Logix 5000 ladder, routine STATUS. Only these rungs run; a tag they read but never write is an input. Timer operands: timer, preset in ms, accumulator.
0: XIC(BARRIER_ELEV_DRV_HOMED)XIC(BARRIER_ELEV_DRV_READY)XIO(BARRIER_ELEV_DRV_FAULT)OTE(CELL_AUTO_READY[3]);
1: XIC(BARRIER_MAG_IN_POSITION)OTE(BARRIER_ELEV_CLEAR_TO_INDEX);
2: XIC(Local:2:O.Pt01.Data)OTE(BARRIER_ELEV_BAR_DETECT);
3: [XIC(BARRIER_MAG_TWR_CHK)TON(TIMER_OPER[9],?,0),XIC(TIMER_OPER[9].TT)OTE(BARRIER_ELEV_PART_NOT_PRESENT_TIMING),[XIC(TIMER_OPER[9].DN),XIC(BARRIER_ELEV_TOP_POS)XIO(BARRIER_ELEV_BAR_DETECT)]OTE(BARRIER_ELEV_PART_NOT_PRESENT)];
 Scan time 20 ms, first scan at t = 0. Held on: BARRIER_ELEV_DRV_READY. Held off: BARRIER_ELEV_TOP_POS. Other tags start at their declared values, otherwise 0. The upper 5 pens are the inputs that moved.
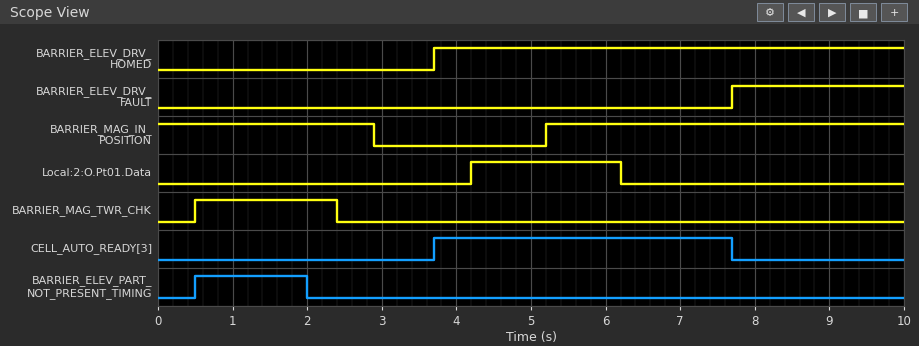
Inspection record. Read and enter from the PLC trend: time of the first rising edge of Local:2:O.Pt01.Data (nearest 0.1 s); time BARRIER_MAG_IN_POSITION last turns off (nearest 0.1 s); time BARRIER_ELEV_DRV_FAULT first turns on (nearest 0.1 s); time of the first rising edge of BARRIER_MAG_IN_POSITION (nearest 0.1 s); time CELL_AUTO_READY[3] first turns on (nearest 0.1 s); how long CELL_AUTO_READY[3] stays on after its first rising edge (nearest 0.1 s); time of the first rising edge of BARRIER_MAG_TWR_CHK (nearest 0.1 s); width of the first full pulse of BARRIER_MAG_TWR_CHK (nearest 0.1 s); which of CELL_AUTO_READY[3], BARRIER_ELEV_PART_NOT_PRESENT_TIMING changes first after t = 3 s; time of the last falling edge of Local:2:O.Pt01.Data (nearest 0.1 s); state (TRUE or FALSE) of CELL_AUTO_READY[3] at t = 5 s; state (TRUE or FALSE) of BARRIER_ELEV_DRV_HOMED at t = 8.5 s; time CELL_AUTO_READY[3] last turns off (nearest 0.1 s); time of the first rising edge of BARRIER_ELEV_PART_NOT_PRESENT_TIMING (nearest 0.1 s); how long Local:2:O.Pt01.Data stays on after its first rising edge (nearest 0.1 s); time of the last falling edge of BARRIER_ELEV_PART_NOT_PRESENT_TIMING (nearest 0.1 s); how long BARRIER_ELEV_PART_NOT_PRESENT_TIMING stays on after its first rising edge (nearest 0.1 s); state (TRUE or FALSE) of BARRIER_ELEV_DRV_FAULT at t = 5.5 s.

4.2 s
2.9 s
7.7 s
5.2 s
3.7 s
4.0 s
0.5 s
1.9 s
CELL_AUTO_READY[3]
6.2 s
TRUE
TRUE
7.7 s
0.5 s
2.0 s
2.0 s
1.5 s
FALSE
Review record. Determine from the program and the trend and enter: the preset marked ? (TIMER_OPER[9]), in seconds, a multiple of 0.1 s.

1.5 s
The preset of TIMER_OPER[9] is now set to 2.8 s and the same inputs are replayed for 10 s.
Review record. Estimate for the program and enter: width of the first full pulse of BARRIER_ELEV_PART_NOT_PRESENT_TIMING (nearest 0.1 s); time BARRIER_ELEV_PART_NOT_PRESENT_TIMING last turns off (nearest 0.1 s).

1.9 s
2.4 s
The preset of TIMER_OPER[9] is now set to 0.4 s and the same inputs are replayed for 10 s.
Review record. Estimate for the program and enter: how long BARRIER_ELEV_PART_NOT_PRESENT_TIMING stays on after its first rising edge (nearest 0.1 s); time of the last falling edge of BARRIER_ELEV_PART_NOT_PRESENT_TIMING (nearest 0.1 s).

0.4 s
0.9 s
